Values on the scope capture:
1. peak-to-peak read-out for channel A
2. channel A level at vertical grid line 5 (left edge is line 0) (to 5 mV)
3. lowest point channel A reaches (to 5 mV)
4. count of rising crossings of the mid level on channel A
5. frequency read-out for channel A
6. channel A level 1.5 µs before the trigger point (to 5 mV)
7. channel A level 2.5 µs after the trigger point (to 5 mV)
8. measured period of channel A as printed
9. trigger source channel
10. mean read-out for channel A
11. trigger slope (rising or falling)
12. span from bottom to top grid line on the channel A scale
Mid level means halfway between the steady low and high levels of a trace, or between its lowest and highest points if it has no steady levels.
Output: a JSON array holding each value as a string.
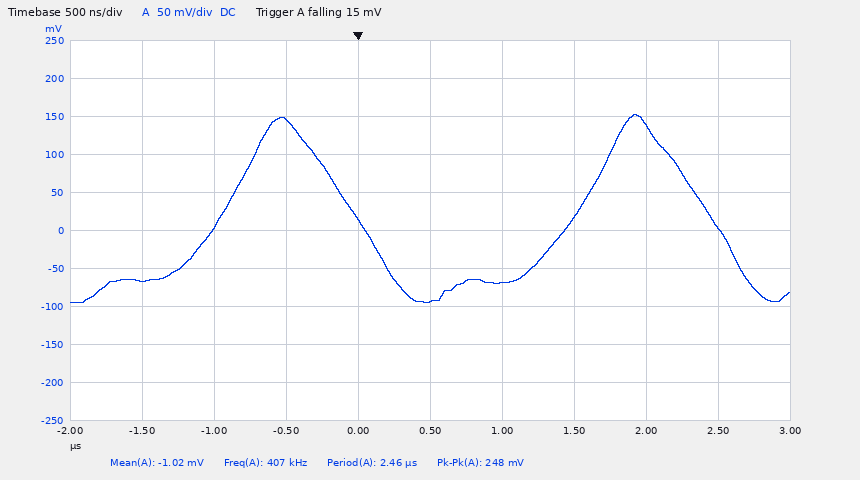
["248 mV", "-95 mV", "-95 mV", "2", "407 kHz", "-65 mV", "5 mV", "2.46 µs", "channel A", "-1.02 mV", "falling", "500 mV"]
